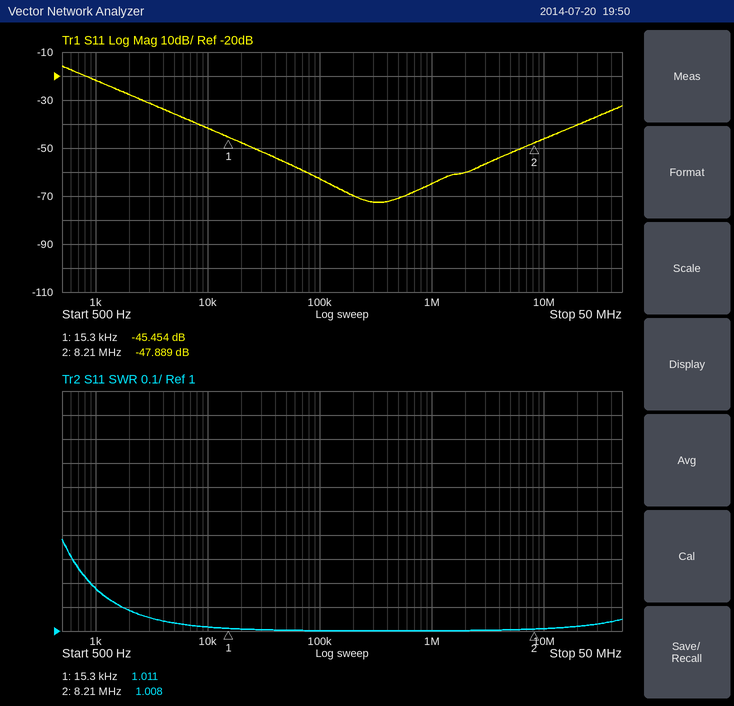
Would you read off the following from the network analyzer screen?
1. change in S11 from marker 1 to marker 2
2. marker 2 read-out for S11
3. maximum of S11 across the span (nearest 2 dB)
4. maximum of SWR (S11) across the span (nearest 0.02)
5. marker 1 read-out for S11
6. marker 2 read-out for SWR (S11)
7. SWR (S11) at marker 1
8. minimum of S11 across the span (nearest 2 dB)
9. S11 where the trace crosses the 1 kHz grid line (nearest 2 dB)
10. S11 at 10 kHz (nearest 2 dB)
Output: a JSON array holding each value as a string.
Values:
["-2.435 dB", "-47.889 dB", "-16 dB", "1.38", "-45.454 dB", "1.008", "1.011", "-72 dB", "-22 dB", "-42 dB"]
